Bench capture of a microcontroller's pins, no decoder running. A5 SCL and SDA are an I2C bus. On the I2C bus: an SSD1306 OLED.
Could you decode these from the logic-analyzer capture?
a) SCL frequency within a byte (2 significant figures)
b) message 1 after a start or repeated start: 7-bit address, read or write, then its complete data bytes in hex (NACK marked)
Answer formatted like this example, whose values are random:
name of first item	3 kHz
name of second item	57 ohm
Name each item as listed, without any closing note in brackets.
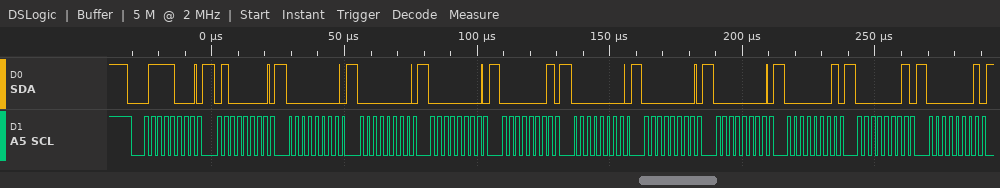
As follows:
SCL frequency within a byte	400 kHz
message 1 after a start or repeated start: 7-bit address, read or write, then its complete data bytes in hex	0x3C write: 40 00 00 00 01 00 00 00 01 01 01
